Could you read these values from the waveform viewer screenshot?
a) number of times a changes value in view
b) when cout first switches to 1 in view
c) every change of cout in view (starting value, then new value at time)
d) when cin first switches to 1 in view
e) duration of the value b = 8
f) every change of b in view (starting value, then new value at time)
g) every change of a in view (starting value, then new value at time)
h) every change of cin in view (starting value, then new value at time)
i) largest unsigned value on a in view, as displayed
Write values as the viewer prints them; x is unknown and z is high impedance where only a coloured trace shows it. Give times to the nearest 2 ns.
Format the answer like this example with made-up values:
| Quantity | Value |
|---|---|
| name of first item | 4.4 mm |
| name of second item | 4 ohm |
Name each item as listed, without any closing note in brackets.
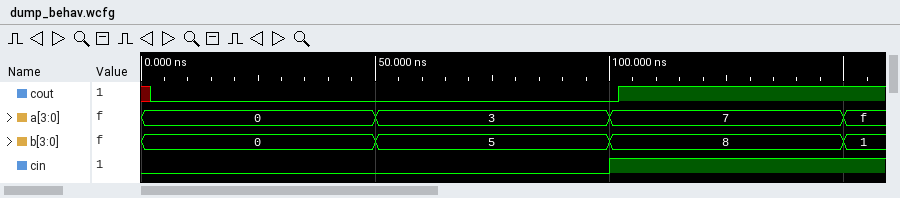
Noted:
| Quantity | Value |
|---|---|
| number of times a changes value in view | 3 |
| when cout first switches to 1 in view | 102 ns |
| every change of cout in view | x, 0 at 2 ns, 1 at 102 ns |
| when cin first switches to 1 in view | 100 ns |
| duration of the value b = 8 | 50 ns |
| every change of b in view | 0, 5 at 50 ns, 8 at 100 ns, 1 at 150 ns |
| every change of a in view | 0, 3 at 50 ns, 7 at 100 ns, f at 150 ns |
| every change of cin in view | 0, 1 at 100 ns |
| largest unsigned value on a in view, as displayed | f |
